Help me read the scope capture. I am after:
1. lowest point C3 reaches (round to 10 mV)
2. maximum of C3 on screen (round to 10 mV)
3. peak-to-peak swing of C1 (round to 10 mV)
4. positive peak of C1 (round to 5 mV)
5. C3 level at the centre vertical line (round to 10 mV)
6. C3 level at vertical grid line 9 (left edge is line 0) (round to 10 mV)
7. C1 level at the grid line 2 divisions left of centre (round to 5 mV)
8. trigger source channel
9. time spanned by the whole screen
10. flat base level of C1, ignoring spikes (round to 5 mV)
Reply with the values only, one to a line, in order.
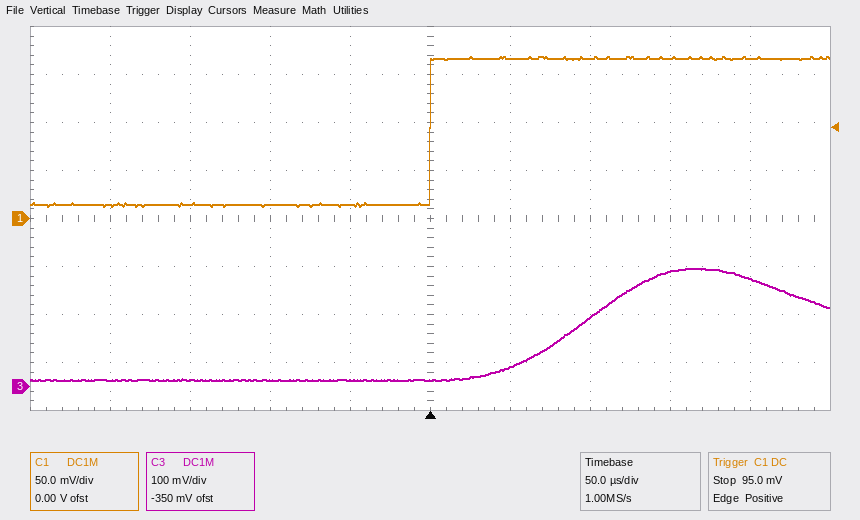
10 mV
250 mV
160 mV
170 mV
10 mV
220 mV
15 mV
C1
500 µs
15 mV
